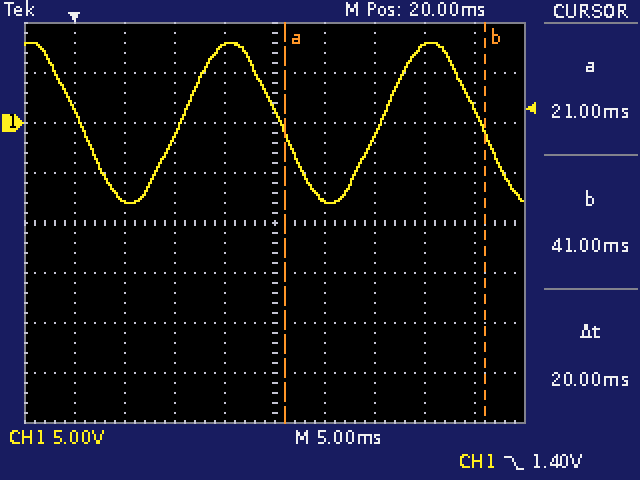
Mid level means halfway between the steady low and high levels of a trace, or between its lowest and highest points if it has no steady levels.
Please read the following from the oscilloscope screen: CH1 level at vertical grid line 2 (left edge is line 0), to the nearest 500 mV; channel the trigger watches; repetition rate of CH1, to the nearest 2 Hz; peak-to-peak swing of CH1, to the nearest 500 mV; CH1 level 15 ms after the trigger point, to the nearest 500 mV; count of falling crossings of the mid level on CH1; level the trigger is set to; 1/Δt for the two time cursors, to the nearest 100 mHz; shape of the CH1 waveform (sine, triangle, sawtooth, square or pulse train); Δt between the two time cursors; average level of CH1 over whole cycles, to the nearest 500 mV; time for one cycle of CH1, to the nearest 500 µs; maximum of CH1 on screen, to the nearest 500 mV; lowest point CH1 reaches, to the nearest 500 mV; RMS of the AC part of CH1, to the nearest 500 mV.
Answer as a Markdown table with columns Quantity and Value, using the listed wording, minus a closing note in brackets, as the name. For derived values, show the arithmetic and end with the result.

| Quantity | Value |
|---|---|
| CH1 level at vertical grid line 2 (left edge is line 0), to the nearest 500 mV | -8.0 V |
| channel the trigger watches | CH1 |
| repetition rate of CH1, to the nearest 2 Hz | 1 / 20.0 ms ≈ 50 Hz |
| peak-to-peak swing of CH1, to the nearest 500 mV | 8.0 V − (-8.0 V) = 16.0 V |
| CH1 level 15 ms after the trigger point, to the nearest 500 mV | 8.0 V |
| count of falling crossings of the mid level on CH1 | 3 |
| level the trigger is set to | 1.40 V |
| 1/Δt for the two time cursors, to the nearest 100 mHz | 1 / 20 ms ≈ 50.0 Hz |
| shape of the CH1 waveform | sine |
| Δt between the two time cursors | 20 ms |
| average level of CH1 over whole cycles, to the nearest 500 mV | (8.0 V + (-8.0 V)) / 2 ≈ 0.0 V |
| time for one cycle of CH1, to the nearest 500 µs | 20.0 ms |
| maximum of CH1 on screen, to the nearest 500 mV | 8.0 V |
| lowest point CH1 reaches, to the nearest 500 mV | -8.0 V |
| RMS of the AC part of CH1, to the nearest 500 mV | 16.0 V / (2√2) ≈ 5.66 V, so 5.5 V to the nearest 500 mV |
